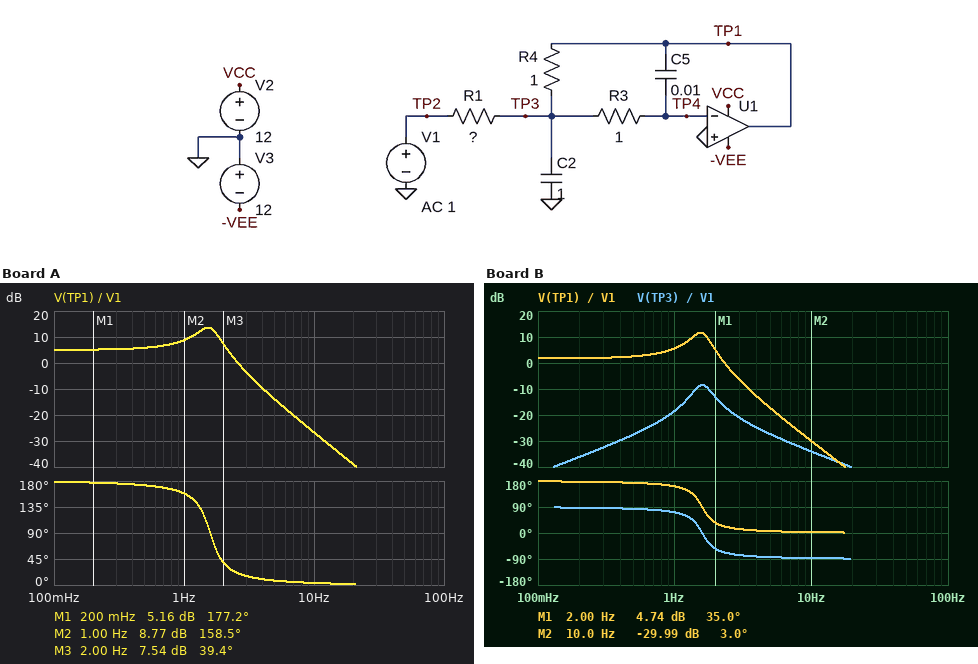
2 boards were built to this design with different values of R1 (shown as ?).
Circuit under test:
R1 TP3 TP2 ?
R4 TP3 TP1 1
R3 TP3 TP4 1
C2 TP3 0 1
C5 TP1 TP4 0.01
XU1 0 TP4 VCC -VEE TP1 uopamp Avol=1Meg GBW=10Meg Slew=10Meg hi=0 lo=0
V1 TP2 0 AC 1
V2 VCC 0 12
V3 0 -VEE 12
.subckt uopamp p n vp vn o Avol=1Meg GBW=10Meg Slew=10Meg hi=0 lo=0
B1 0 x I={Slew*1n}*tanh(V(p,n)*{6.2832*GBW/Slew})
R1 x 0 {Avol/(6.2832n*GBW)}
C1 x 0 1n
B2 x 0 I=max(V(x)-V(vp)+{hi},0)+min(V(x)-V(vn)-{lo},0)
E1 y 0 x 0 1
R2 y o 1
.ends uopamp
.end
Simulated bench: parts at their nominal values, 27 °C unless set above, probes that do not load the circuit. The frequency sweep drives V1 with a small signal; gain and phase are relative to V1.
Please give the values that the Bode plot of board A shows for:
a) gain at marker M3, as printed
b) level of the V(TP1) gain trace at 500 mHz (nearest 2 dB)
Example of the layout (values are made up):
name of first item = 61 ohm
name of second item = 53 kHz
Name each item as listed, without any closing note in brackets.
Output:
gain at marker M3, as printed = 7.54 dB
level of the V(TP1) gain trace at 500 mHz = 6 dB
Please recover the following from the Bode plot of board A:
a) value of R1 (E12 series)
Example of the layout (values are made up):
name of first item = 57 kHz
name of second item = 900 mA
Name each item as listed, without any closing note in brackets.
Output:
value of R1 = 0.56 Ω
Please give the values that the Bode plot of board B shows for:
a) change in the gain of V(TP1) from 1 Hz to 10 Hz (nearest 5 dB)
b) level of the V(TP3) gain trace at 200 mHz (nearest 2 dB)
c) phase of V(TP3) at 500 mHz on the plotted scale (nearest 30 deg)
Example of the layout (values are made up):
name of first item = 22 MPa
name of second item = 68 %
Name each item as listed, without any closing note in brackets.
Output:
change in the gain of V(TP1) from 1 Hz to 10 Hz = -35 dB
level of the V(TP3) gain trace at 200 mHz = -36 dB
phase of V(TP3) at 500 mHz on the plotted scale = 90 deg
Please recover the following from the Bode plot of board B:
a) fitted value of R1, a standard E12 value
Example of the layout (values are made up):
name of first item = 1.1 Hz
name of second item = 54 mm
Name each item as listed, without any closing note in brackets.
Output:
fitted value of R1, a standard E12 value = 0.82 Ω
